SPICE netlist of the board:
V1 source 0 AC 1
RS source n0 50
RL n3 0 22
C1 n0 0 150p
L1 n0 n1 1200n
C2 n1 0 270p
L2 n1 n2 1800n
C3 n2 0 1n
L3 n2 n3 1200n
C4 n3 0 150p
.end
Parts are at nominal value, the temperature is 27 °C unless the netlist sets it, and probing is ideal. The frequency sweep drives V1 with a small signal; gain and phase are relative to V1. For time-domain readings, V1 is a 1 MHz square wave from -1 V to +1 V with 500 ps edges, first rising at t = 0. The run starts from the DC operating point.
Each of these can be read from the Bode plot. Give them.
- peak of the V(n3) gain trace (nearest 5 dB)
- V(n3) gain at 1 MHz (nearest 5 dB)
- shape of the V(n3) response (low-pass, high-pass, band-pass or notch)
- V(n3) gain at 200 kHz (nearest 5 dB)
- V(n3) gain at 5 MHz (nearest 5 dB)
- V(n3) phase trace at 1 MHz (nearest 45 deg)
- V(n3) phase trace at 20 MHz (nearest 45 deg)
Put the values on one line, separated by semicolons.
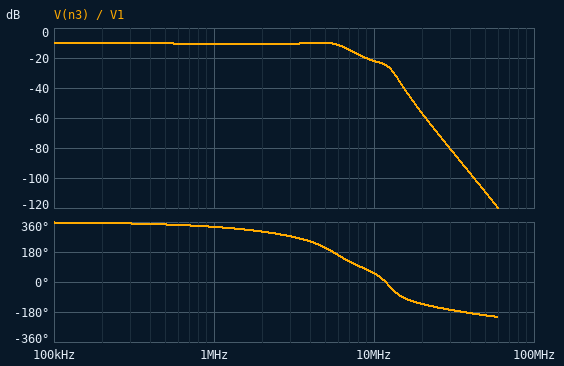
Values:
-10 dB; -10 dB; low-pass; -10 dB; -10 dB; 315 deg; -135 deg
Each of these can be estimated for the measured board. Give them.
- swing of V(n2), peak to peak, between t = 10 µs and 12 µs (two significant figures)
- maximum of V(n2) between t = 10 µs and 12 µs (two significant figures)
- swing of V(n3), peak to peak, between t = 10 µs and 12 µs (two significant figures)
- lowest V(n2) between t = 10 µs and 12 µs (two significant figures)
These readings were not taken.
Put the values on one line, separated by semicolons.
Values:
1.3 V; 640 mV; 730 mV; -640 mV
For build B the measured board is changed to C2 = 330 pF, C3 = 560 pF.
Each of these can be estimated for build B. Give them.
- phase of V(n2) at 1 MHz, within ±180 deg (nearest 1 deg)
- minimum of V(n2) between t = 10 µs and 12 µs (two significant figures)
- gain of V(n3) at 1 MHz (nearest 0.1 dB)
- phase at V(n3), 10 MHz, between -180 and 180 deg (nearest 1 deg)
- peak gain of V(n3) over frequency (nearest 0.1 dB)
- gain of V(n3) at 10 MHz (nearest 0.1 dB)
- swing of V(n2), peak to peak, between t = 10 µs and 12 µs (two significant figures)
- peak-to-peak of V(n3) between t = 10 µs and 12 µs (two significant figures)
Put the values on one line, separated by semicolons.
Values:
-8 deg; -810 mV; -10.5 dB; 59 deg; -9.6 dB; -13.4 dB; 1.6 V; 760 mV
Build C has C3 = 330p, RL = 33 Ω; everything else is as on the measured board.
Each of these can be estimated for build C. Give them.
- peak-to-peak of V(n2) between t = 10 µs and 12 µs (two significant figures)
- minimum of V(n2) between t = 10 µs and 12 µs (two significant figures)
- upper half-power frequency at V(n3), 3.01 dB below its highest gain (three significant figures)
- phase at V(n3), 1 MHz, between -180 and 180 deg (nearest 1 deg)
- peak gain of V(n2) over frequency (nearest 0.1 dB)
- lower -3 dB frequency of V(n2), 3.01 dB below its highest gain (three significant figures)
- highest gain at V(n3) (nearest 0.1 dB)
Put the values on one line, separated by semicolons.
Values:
1.7 V; -850 mV; 13.5 MHz; -24 deg; 0.3 dB; 7.81 MHz; -7.8 dB
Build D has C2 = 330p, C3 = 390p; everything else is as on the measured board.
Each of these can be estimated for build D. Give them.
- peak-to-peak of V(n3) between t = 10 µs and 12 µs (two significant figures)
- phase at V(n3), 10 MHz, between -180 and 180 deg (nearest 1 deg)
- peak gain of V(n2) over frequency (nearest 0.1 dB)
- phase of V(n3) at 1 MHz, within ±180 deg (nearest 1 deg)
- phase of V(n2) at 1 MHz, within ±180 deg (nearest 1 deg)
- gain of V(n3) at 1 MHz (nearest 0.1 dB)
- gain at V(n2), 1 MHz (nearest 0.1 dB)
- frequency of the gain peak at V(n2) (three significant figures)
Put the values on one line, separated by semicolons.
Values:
730 mV; 93 deg; 0.8 dB; -26 deg; -7 deg; -10.5 dB; -10.1 dB; 11.2 MHz
